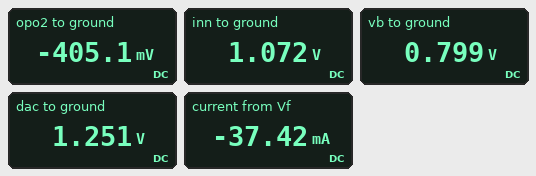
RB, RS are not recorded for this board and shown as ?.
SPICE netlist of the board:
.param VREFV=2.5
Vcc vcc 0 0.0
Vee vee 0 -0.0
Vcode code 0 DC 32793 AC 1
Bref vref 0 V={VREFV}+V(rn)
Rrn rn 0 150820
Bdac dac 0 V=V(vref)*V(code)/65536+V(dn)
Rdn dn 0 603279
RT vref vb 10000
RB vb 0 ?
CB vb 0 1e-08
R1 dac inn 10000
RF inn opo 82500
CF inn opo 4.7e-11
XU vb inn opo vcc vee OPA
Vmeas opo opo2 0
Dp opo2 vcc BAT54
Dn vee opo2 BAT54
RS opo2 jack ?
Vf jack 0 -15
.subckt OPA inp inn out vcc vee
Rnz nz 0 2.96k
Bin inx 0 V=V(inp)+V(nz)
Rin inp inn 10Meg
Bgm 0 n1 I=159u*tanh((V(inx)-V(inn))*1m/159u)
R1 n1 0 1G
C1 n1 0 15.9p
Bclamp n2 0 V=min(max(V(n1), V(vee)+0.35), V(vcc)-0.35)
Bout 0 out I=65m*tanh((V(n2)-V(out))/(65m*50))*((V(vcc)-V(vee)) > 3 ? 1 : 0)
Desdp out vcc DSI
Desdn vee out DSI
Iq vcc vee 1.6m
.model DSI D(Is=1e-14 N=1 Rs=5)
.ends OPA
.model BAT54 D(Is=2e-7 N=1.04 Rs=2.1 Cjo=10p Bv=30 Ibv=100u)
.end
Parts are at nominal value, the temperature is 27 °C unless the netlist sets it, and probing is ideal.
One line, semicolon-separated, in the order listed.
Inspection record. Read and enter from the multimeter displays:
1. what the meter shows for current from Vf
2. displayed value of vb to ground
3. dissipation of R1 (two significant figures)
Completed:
-37.42 mA; 0.799 V; 3.2 µW
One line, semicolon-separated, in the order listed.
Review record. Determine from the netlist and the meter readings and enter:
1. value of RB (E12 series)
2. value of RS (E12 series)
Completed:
4.7 kΩ; 390 Ω
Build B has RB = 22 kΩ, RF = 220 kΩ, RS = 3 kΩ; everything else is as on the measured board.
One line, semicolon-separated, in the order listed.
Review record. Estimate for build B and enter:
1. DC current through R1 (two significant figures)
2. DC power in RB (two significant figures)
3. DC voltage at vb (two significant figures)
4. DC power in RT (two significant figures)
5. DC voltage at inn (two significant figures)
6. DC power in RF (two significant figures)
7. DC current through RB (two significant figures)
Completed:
6.6 µA; 130 µW; 1.7 V; 61 µW; 1.2 V; 9.8 µW; 78 µA
